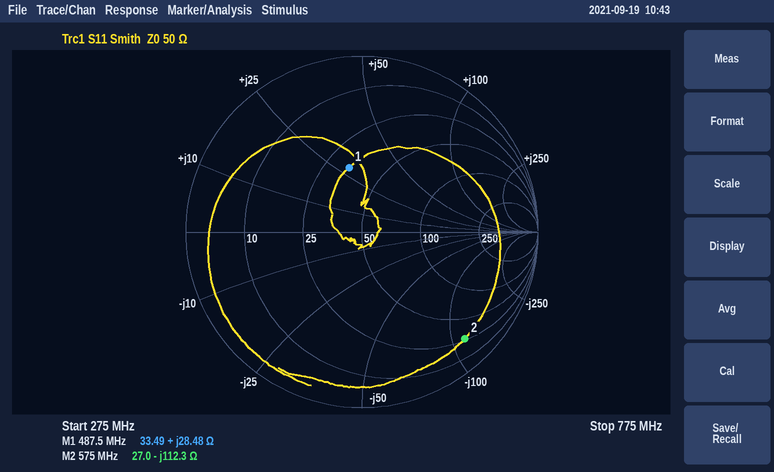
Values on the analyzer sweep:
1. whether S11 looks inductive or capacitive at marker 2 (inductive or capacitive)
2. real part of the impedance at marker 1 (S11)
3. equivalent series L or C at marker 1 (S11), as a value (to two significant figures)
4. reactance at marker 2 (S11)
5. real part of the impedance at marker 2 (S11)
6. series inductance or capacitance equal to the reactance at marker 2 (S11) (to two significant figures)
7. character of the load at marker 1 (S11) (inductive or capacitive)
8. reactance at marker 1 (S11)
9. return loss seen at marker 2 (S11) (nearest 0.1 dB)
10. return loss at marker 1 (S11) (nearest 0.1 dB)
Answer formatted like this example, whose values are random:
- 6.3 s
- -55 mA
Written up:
- capacitive
- 33.49 Ω
- 9.3 nH
- -112.3 Ω
- 27.0 Ω
- 2.5 pF
- inductive
- +28.48 Ω
- 1.5 dB
- 8.6 dB
